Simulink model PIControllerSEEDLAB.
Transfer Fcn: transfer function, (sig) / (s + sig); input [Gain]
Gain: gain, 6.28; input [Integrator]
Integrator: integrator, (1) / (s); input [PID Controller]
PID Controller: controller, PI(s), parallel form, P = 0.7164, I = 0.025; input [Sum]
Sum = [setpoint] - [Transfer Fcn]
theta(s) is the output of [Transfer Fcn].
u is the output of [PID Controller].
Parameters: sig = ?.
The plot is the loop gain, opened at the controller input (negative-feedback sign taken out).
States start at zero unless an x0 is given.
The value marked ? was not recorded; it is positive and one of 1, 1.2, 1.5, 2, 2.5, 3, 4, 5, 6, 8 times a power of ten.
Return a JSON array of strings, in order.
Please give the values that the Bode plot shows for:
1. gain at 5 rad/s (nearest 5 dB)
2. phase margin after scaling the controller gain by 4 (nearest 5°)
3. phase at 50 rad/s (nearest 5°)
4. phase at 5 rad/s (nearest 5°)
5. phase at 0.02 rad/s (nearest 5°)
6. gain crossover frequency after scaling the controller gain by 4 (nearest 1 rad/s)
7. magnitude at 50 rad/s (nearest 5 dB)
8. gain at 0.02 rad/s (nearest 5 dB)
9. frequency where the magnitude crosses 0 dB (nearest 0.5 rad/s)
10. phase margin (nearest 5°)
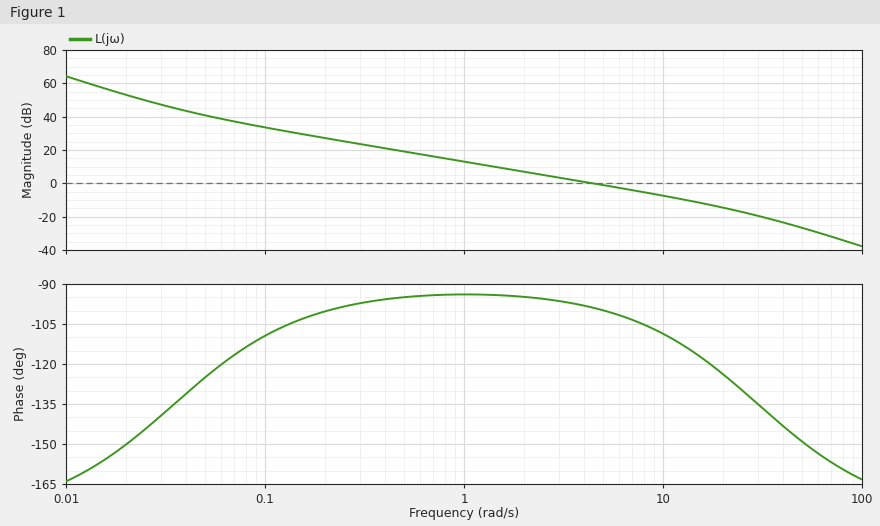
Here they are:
["0 dB", "60°", "-150°", "-100°", "-150°", "16 rad/s", "-25 dB", "55 dB", "4.5 rad/s", "80°"]
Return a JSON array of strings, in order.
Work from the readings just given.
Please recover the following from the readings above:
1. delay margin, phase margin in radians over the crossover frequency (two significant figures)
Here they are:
["0.31 s"]
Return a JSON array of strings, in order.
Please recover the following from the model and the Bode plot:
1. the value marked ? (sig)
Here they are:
["30"]
